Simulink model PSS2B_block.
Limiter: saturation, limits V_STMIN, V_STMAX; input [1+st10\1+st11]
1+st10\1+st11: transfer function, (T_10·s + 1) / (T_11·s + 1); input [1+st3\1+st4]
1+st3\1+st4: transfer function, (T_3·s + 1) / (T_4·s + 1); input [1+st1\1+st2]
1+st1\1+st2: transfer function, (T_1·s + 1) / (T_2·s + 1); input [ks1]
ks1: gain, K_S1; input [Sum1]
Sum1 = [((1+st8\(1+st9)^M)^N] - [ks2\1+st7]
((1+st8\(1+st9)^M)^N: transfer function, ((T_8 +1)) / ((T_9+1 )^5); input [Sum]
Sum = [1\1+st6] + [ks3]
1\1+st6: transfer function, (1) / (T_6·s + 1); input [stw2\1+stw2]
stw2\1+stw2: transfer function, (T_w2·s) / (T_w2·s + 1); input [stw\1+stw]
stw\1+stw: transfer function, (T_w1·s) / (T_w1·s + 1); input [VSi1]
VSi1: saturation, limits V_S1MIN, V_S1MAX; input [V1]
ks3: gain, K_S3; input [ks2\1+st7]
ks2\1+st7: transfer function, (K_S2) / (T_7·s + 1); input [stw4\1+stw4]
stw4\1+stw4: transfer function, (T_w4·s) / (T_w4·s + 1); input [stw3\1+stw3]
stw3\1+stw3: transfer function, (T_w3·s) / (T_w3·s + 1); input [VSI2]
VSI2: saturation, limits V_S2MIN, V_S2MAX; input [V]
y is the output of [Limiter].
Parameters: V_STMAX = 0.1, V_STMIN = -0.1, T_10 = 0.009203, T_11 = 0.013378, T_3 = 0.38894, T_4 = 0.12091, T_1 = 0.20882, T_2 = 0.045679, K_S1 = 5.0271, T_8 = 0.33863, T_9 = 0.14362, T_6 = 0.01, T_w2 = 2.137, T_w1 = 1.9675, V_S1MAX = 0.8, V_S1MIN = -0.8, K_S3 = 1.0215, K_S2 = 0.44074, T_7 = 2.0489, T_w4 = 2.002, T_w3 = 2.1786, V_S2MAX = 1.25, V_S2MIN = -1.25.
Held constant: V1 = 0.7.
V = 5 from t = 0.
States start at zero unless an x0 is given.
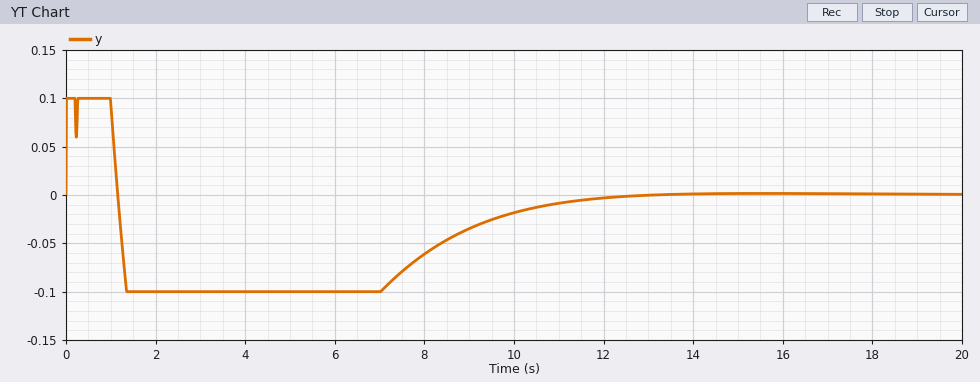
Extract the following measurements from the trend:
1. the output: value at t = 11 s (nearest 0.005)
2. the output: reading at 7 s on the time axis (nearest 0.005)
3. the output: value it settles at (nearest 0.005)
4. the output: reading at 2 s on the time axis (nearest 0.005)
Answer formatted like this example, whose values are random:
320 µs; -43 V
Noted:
-0.010; -0.100; 0.000; -0.100
